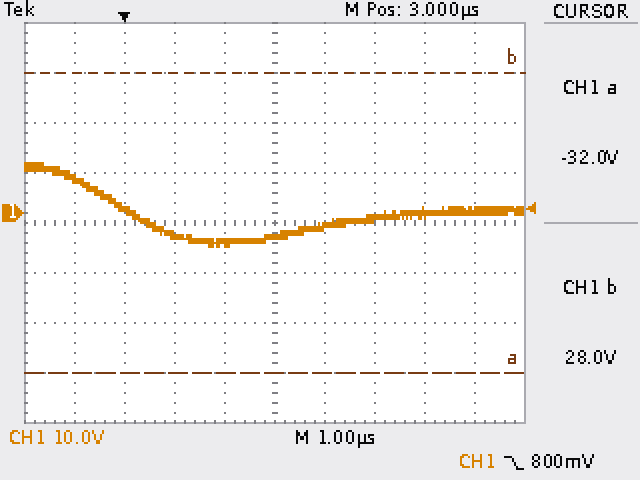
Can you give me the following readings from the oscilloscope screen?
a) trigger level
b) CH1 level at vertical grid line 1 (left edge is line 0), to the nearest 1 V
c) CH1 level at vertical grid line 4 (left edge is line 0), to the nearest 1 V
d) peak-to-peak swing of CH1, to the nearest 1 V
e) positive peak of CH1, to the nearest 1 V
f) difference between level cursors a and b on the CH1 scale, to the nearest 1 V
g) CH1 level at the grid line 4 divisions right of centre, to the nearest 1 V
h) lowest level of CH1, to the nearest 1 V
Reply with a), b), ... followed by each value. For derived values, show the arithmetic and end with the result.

a) 800 mV
b) 7 V
c) -6 V
d) 10 V − (-7 V) = 17 V
e) 10 V
f) 60 V
g) 0 V
h) -7 V
